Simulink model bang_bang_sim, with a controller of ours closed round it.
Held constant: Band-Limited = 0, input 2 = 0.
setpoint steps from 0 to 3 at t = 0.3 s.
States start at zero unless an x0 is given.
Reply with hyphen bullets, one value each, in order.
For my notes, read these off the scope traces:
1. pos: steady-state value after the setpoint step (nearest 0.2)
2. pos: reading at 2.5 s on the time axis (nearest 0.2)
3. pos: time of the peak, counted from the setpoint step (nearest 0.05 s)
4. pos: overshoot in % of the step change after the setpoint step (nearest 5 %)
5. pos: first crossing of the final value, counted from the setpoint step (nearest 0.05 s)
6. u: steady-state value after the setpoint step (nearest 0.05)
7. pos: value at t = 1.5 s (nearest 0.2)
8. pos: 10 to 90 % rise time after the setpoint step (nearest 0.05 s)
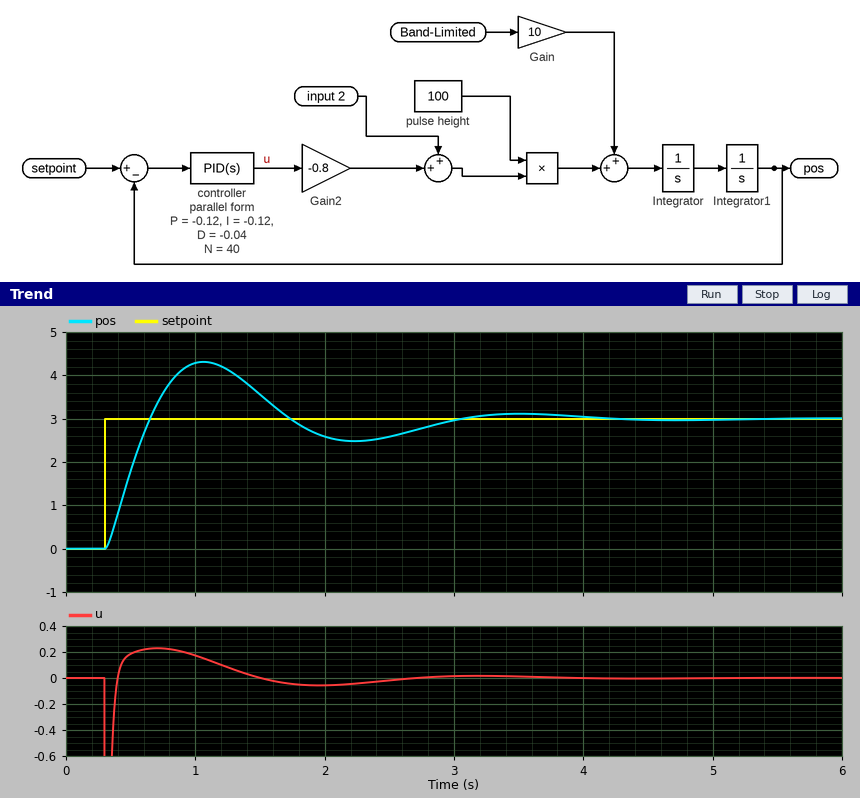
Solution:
- 3.0
- 2.6
- 0.75 s
- 45 %
- 0.35 s
- 0.00
- 3.6
- 0.25 s
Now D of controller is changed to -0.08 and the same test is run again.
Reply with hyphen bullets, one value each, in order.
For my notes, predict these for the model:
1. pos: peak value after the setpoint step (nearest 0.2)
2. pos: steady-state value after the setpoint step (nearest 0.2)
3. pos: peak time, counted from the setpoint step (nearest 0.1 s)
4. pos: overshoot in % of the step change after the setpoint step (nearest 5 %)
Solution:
- 3.6
- 3.0
- 0.6 s
- 20 %
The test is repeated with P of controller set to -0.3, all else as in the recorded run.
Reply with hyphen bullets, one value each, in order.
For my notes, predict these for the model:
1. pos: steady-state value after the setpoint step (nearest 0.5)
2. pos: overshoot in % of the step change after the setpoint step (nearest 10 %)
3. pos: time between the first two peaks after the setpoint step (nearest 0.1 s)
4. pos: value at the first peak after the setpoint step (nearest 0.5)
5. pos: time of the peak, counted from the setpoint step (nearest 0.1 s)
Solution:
- 3.0
- 50 %
- 1.3 s
- 4.5
- 0.5 s
